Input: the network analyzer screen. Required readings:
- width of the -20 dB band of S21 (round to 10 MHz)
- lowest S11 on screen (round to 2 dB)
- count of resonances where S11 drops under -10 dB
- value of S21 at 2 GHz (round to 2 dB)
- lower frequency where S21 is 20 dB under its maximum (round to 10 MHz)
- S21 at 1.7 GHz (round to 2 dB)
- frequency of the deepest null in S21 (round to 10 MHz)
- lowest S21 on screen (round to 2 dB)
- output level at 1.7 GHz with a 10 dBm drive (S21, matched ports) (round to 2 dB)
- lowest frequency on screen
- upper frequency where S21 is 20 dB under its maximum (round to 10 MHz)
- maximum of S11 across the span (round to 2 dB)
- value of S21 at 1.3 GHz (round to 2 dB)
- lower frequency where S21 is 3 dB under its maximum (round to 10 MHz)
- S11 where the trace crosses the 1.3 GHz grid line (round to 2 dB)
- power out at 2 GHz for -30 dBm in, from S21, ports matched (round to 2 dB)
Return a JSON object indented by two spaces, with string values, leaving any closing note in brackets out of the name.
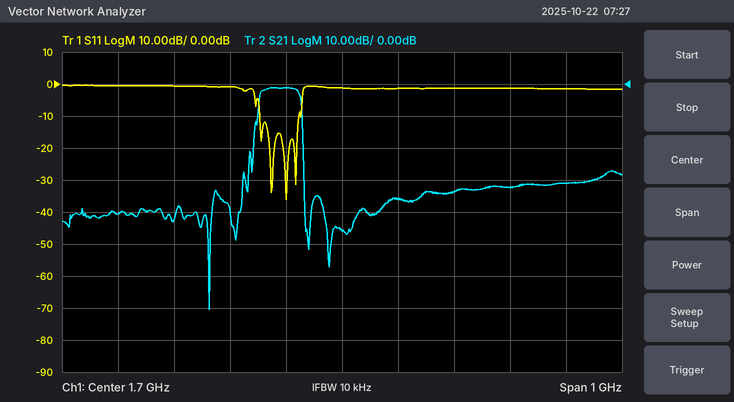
{
  "width of the -20 dB band of S21": "90 MHz",
  "lowest S11 on screen": "-36 dB",
  "count of resonances where S11 drops under -10 dB": "4",
  "value of S21 at 2 GHz": "-32 dB",
  "lower frequency where S21 is 20 dB under its maximum": "1.54 GHz",
  "S21 at 1.7 GHz": "-46 dB",
  "frequency of the deepest null in S21": "1.46 GHz",
  "lowest S21 on screen": "-70 dB",
  "output level at 1.7 GHz with a 10 dBm drive (S21, matched ports)": "-36 dBm",
  "lowest frequency on screen": "1.2 GHz",
  "upper frequency where S21 is 20 dB under its maximum": "1.63 GHz",
  "maximum of S11 across the span": "0 dB",
  "value of S21 at 1.3 GHz": "-40 dB",
  "lower frequency where S21 is 3 dB under its maximum": "1.55 GHz",
  "S11 where the trace crosses the 1.3 GHz grid line": "0 dB",
  "power out at 2 GHz for -30 dBm in, from S21, ports matched": "-62 dBm"
}
